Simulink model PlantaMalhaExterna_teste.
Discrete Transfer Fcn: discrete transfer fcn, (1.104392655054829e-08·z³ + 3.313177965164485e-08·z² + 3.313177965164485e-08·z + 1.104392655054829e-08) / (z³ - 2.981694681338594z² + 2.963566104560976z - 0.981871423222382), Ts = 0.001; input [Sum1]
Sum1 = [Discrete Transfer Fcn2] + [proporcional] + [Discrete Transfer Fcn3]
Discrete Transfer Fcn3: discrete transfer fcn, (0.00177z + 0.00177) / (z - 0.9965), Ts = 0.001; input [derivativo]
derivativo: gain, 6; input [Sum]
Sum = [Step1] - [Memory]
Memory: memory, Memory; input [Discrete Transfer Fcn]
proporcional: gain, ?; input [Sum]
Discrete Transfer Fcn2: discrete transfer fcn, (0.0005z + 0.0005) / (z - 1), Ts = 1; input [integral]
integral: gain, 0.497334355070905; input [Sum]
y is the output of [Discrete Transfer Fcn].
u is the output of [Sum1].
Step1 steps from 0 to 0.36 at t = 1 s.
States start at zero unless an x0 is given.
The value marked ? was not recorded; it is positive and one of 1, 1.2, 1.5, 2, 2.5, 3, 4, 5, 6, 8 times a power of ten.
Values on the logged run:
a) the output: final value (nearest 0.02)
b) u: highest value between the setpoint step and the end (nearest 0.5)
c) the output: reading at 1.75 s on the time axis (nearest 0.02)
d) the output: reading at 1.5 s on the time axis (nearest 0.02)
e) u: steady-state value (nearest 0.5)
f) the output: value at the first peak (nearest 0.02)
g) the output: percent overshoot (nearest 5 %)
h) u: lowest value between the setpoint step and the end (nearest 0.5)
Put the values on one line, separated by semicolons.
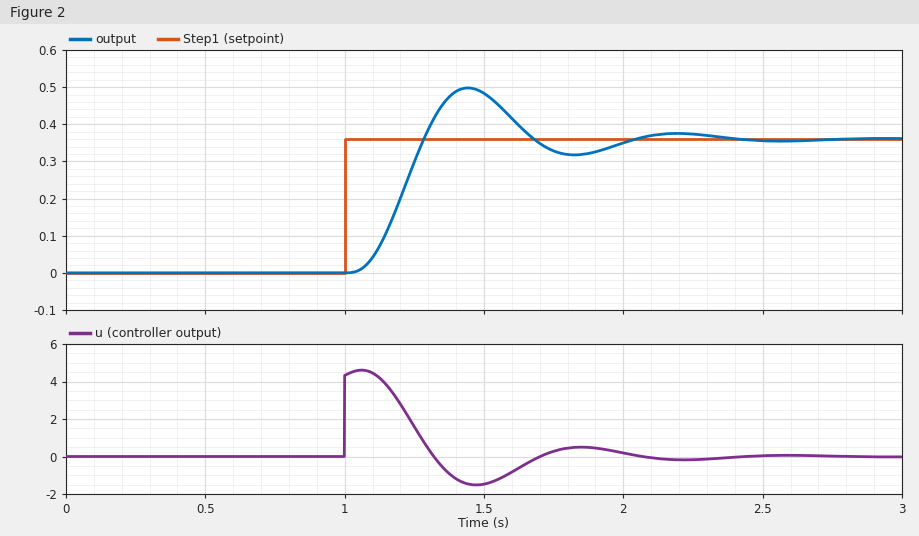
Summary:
0.36; 4.5; 0.32; 0.48; 0.0; 0.50; 40 %; -1.5
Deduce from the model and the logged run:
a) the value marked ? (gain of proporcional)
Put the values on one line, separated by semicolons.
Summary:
12
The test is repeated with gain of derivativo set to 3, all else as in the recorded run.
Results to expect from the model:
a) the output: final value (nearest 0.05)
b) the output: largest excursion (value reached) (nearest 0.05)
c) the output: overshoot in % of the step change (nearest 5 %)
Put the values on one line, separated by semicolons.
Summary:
0.35; 0.45; 30 %
